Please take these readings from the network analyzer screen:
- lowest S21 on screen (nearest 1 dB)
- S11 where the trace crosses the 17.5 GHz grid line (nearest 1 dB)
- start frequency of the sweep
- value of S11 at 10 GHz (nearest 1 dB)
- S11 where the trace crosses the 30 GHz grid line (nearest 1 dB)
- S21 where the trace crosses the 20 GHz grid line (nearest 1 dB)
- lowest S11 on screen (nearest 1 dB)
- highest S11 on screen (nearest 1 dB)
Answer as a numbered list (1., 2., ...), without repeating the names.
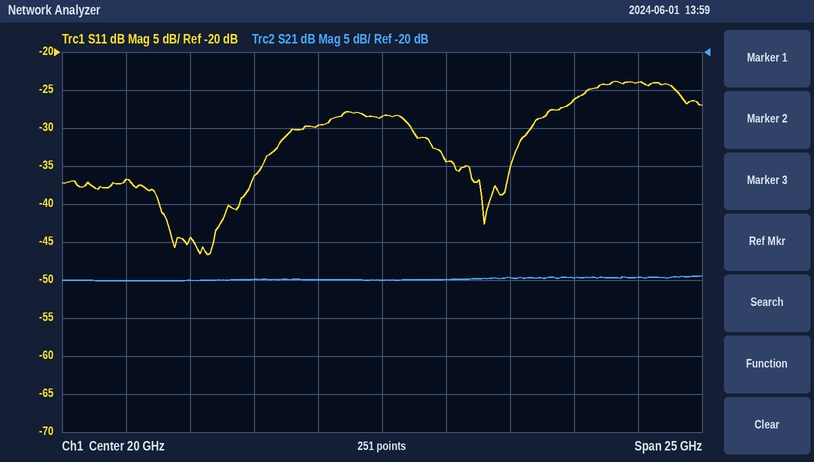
1. -50 dB
2. -30 dB
3. 7.5 GHz
4. -37 dB
5. -24 dB
6. -50 dB
7. -47 dB
8. -24 dB
